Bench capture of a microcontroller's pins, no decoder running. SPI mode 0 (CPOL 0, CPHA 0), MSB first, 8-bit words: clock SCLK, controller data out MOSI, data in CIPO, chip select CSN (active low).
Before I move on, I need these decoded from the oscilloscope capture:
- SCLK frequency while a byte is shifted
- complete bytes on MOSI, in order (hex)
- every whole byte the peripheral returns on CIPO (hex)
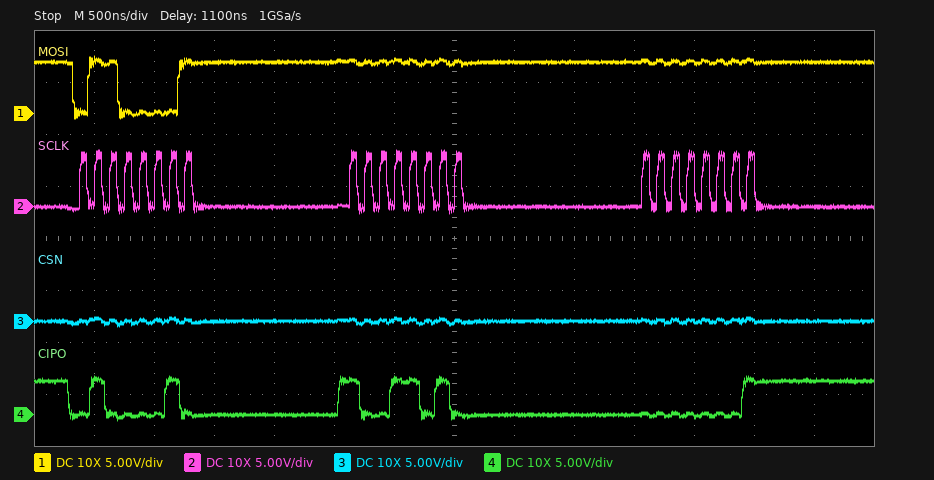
8 MHz
61 FF FF
42 9A 01
